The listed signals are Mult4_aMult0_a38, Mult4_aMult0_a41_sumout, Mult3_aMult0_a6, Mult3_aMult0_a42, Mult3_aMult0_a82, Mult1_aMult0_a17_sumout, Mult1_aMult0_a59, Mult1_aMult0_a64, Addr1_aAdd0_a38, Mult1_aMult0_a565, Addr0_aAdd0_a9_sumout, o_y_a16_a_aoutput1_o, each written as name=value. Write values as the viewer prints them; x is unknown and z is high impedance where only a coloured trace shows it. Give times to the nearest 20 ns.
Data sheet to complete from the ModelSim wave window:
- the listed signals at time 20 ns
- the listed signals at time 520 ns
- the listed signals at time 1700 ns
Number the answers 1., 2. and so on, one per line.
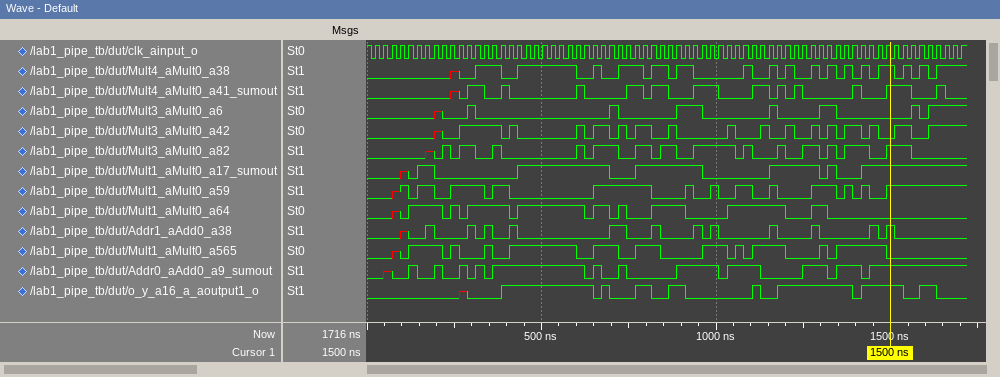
1. Mult4_aMult0_a38=0, Mult4_aMult0_a41_sumout=0, Mult3_aMult0_a6=0, Mult3_aMult0_a42=0, Mult3_aMult0_a82=0, Mult1_aMult0_a17_sumout=0, Mult1_aMult0_a59=0, Mult1_aMult0_a64=0, Addr1_aAdd0_a38=0, Mult1_aMult0_a565=0, Addr0_aAdd0_a9_sumout=0, o_y_a16_a_aoutput1_o=0
2. Mult4_aMult0_a38=1, Mult4_aMult0_a41_sumout=0, Mult3_aMult0_a6=0, Mult3_aMult0_a42=0, Mult3_aMult0_a82=0, Mult1_aMult0_a17_sumout=1, Mult1_aMult0_a59=0, Mult1_aMult0_a64=1, Addr1_aAdd0_a38=0, Mult1_aMult0_a565=1, Addr0_aAdd0_a9_sumout=1, o_y_a16_a_aoutput1_o=1
3. Mult4_aMult0_a38=1, Mult4_aMult0_a41_sumout=0, Mult3_aMult0_a6=1, Mult3_aMult0_a42=1, Mult3_aMult0_a82=0, Mult1_aMult0_a17_sumout=1, Mult1_aMult0_a59=1, Mult1_aMult0_a64=0, Addr1_aAdd0_a38=0, Mult1_aMult0_a565=0, Addr0_aAdd0_a9_sumout=1, o_y_a16_a_aoutput1_o=0
